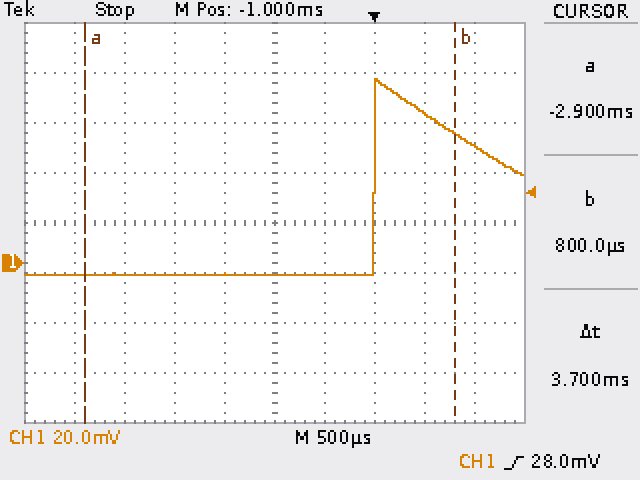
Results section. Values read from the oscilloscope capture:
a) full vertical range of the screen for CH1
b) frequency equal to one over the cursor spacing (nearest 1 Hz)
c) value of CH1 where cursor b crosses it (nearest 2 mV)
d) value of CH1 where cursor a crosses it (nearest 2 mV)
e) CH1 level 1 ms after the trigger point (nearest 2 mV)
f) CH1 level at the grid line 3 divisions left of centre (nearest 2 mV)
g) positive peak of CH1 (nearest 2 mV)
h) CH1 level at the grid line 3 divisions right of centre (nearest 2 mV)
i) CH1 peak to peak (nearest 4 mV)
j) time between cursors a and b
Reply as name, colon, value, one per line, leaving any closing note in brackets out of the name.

full vertical range of the screen for CH1: 160 mV
frequency equal to one over the cursor spacing: 270 Hz
value of CH1 where cursor b crosses it: 52 mV
value of CH1 where cursor a crosses it: -4 mV
CH1 level 1 ms after the trigger point: 46 mV
CH1 level at the grid line 3 divisions left of centre: -4 mV
positive peak of CH1: 74 mV
CH1 level at the grid line 3 divisions right of centre: 60 mV
CH1 peak to peak: 80 mV
time between cursors a and b: 3.7 ms
